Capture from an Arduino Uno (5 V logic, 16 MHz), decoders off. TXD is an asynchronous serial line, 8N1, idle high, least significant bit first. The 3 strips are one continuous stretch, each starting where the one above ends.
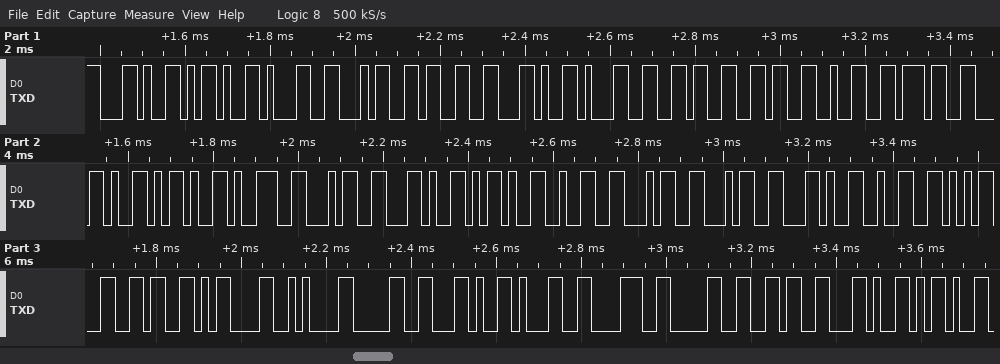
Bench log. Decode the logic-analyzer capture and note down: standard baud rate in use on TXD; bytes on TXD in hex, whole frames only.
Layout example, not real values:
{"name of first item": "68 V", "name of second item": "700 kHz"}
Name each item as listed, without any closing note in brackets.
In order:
{"standard baud rate in use on TXD": "57600 baud", "bytes on TXD in hex, whole frames only": "2C 2D 31 34 33 2C 31 36 36 32 37 2C 2D 39 34 2C 2D 32 34 34 2C 32 35 36 0D 0A 30 2C 31 38 30 36 2C 2D"}
